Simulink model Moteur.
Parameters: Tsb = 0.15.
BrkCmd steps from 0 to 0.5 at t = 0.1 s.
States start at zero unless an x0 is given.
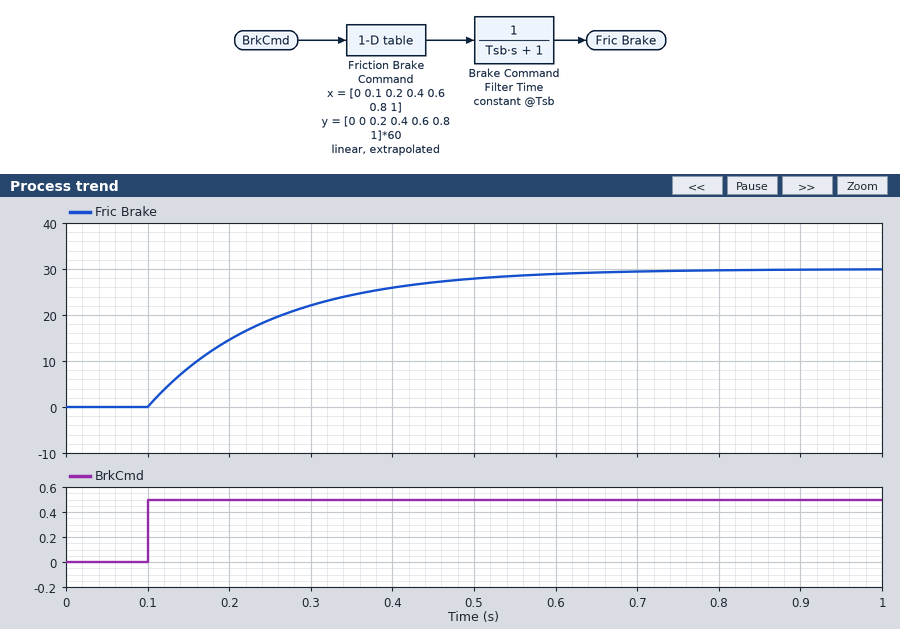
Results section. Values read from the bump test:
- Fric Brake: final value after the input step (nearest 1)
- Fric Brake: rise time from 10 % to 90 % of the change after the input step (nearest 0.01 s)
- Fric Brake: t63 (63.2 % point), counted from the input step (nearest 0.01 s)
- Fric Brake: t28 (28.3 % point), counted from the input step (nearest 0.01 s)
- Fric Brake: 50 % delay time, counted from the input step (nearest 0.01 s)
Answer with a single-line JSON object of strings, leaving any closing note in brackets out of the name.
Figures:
{"Fric Brake: final value after the input step": "30", "Fric Brake: rise time from 10 % to 90 % of the change after the input step": "0.33 s", "Fric Brake: t63 (63.2 % point), counted from the input step": "0.15 s", "Fric Brake: t28 (28.3 % point), counted from the input step": "0.05 s", "Fric Brake: 50 % delay time, counted from the input step": "0.10 s"}
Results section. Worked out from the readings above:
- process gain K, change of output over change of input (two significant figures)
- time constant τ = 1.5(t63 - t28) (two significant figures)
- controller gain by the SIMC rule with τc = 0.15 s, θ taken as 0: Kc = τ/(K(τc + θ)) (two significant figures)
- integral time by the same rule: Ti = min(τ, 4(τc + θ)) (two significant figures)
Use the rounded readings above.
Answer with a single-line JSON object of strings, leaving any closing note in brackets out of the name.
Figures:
{"process gain K, change of output over change of input": "60", "time constant τ = 1.5(t63 - t28)": "0.15 s", "controller gain by the SIMC rule with τc = 0.15 s, θ taken as 0: Kc = τ/(K(τc + θ))": "0.017", "integral time by the same rule: Ti = min(τ, 4(τc + θ))": "0.15 s"}
